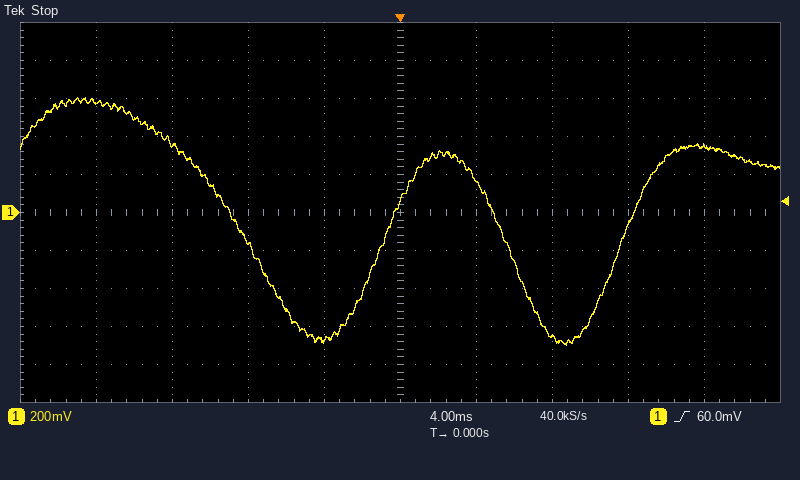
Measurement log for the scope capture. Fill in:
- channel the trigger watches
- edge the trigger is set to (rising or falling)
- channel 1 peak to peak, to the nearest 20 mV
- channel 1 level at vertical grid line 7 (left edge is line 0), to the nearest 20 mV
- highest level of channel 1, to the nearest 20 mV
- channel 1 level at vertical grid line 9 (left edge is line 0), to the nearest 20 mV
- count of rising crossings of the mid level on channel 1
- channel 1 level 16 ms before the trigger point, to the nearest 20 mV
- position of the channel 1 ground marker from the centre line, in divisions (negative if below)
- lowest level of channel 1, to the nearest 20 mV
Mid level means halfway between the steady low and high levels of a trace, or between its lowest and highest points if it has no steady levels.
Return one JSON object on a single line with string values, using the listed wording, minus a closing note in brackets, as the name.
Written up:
{"channel the trigger watches": "channel 1", "edge the trigger is set to": "rising", "channel 1 peak to peak, to the nearest 20 mV": "1.30 V", "channel 1 level at vertical grid line 7 (left edge is line 0), to the nearest 20 mV": "-660 mV", "highest level of channel 1, to the nearest 20 mV": "600 mV", "channel 1 level at vertical grid line 9 (left edge is line 0), to the nearest 20 mV": "340 mV", "count of rising crossings of the mid level on channel 1": "2", "channel 1 level 16 ms before the trigger point, to the nearest 20 mV": "580 mV", "position of the channel 1 ground marker from the centre line, in divisions": "0.0 div", "lowest level of channel 1, to the nearest 20 mV": "-700 mV"}
